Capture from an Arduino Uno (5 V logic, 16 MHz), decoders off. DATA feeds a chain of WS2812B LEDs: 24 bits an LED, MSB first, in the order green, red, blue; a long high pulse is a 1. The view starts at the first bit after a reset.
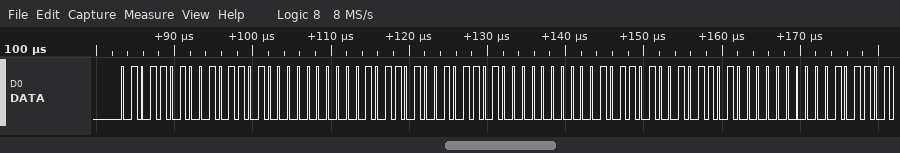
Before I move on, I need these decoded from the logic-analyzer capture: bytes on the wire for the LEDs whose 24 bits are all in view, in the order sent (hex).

5A 5A 00 5A 5A 00 5A 5A 00
